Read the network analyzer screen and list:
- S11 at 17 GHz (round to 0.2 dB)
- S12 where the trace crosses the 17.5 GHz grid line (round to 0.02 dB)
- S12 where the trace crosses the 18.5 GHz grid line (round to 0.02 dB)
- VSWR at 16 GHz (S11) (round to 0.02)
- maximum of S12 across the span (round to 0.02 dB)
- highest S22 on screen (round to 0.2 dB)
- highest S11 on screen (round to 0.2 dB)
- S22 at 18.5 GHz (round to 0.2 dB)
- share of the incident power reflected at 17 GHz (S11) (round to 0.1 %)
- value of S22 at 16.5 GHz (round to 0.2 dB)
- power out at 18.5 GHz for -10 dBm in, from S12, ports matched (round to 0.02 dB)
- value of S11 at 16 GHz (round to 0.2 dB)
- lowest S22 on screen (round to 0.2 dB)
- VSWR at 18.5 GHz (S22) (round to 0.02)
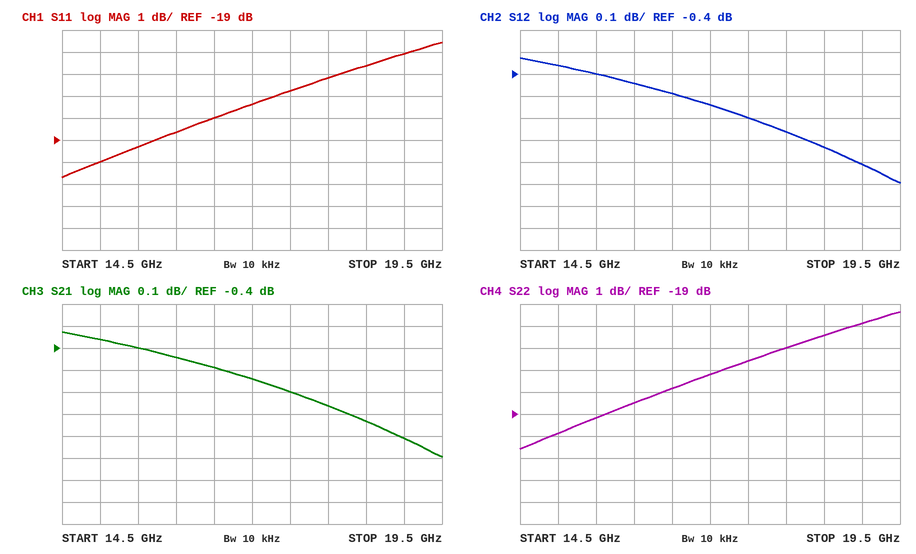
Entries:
-17.4 dB
-0.60 dB
-0.74 dB
1.26
-0.32 dB
-14.4 dB
-14.6 dB
-15.4 dB
1.8 %
-17.8 dB
-10.74 dBm
-18.6 dB
-20.6 dB
1.40
